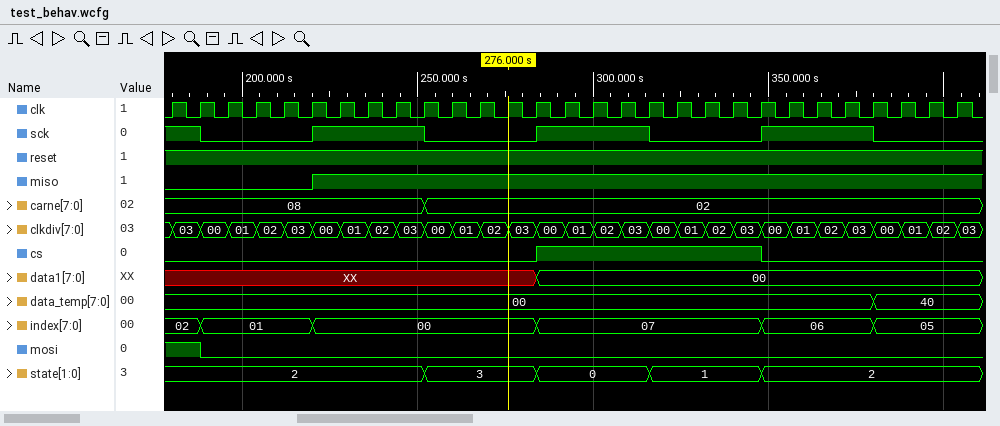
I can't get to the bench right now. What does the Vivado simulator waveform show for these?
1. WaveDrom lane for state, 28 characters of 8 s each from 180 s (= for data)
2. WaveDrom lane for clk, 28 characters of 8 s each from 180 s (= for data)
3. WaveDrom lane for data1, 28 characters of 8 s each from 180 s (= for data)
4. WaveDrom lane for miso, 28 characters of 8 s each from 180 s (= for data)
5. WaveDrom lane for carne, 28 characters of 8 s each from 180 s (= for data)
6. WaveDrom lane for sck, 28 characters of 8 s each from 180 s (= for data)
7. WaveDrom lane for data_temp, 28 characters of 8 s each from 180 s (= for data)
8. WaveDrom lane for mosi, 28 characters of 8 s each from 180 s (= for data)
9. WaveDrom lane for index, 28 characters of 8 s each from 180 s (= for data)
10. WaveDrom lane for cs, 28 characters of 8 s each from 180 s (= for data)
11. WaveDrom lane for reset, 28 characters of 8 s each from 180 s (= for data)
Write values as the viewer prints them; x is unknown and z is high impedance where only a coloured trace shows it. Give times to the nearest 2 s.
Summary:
{name: 'state', wave: '=........=...=...=...=......', data: '2 3 0 1 2'}
{name: 'clk', wave: 'p...........................'}
{name: 'data1', wave: 'x............=..............', data: '00'}
{name: 'miso', wave: '0....1......................'}
{name: 'carne', wave: '=........=..................', data: '08 02'}
{name: 'sck', wave: '10...1...0...1...0...1...0..'}
{name: 'data_temp', wave: '=........................=..', data: '00 40'}
{name: 'mosi', wave: '10..........................'}
{name: 'index', wave: '==...=.......=.......=...=..', data: '02 01 00 07 06 05'}
{name: 'cs', wave: '0............1.......0......'}
{name: 'reset', wave: '1...........................'}
